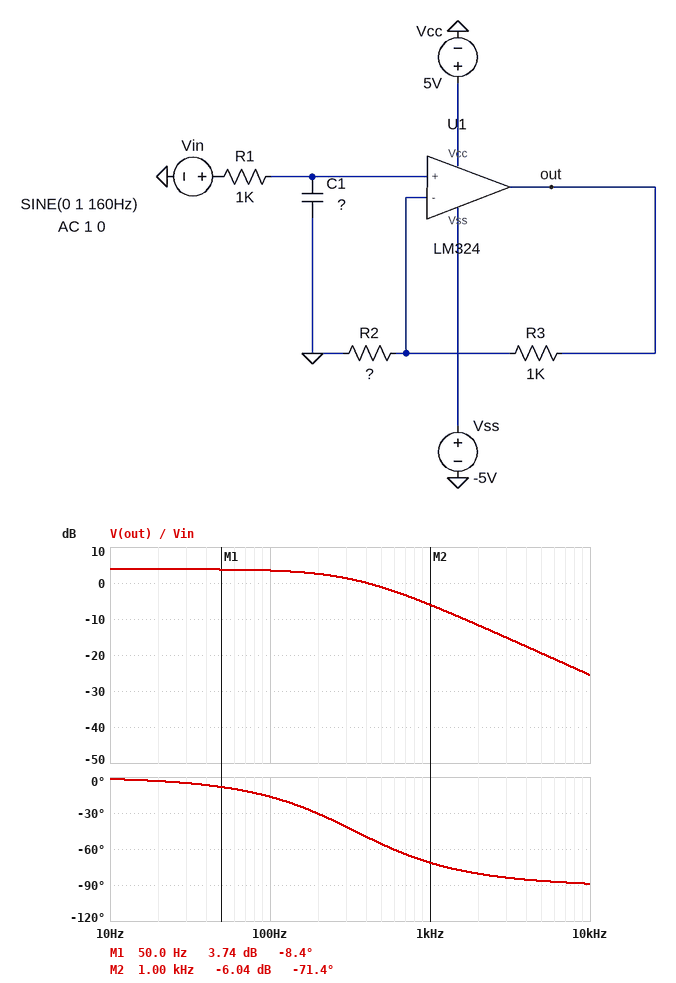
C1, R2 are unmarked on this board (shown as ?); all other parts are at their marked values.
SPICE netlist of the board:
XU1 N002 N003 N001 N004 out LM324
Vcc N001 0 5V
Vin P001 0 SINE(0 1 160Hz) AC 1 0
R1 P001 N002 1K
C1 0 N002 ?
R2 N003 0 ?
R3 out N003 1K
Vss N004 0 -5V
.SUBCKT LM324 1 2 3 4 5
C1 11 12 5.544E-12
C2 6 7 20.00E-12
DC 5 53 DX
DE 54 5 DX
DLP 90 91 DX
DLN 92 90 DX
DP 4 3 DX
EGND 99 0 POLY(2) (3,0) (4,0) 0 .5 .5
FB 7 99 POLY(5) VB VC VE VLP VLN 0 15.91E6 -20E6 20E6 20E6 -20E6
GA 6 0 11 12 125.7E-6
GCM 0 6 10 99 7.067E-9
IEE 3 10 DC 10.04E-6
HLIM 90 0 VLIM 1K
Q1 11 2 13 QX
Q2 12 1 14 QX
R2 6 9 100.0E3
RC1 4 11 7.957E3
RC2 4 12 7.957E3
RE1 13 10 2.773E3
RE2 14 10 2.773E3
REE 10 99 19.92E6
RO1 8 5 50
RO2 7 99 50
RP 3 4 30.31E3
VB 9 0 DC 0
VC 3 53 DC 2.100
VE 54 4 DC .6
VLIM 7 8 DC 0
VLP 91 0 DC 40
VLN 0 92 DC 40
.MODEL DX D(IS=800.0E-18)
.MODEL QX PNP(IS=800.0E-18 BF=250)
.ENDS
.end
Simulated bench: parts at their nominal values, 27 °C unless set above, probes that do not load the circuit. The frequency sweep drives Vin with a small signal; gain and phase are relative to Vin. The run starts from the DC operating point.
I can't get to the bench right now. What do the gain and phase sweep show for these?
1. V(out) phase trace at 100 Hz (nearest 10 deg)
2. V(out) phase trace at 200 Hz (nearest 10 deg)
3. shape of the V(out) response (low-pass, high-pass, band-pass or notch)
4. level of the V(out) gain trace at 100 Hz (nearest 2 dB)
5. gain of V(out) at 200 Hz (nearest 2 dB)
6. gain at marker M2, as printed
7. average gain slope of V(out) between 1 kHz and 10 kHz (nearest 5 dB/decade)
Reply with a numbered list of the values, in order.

1. -20 deg
2. -30 deg
3. low-pass
4. 4 dB
5. 2 dB
6. -6.04 dB
7. -20 dB/decade
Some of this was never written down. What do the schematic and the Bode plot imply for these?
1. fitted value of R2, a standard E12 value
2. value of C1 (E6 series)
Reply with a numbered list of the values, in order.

1. 1.8 kΩ
2. 470 nF
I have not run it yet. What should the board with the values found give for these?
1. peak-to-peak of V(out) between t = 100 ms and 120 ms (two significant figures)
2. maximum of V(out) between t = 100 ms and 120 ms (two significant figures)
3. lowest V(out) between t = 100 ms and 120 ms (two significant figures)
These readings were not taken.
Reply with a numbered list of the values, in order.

1. 2.8 V
2. 1.4 V
3. -1.4 V
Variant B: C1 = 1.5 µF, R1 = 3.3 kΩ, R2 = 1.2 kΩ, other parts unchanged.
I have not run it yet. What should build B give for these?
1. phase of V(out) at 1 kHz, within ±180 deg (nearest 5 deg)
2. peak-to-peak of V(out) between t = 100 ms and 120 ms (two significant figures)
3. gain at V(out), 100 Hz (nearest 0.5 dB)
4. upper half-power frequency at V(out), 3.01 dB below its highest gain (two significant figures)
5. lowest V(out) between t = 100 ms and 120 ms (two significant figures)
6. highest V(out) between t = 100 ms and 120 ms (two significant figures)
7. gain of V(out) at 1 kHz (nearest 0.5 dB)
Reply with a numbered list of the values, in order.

1. -90 deg
2. 720 mV
3. -5.0 dB
4. 32 Hz
5. -360 mV
6. 360 mV
7. -24.5 dB
